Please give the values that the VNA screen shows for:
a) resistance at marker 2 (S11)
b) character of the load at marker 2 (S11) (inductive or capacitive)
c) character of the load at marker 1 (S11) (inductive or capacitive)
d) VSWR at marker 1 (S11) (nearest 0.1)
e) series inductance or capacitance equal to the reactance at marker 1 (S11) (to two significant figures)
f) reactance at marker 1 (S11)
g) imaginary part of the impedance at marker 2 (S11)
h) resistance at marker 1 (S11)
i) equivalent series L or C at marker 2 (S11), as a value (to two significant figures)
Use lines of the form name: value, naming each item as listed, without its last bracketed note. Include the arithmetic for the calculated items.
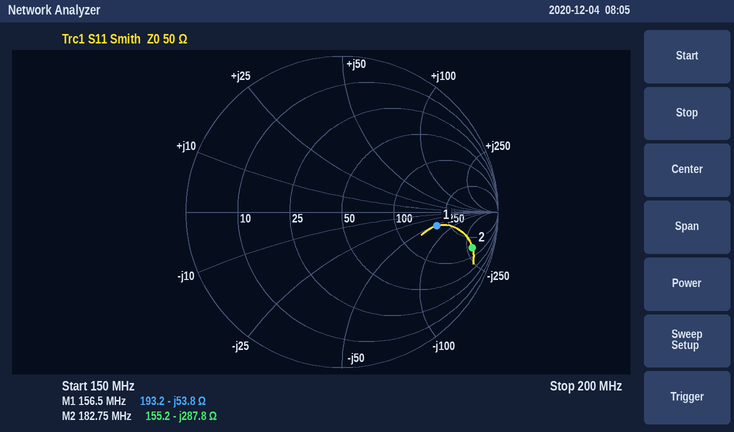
resistance at marker 2: 155.2 Ω
character of the load at marker 2 (S11): capacitive
character of the load at marker 1 (S11): capacitive
VSWR at marker 1 (S11): 4.2
series inductance or capacitance equal to the reactance at marker 1 (S11): C = 1/(2π × 156.5 MHz × 53.8 Ω) ≈ 19 pF
reactance at marker 1: -53.8 Ω
imaginary part of the impedance at marker 2: -287.8 Ω
resistance at marker 1: 193.2 Ω
equivalent series L or C at marker 2 (S11), as a value: C = 1/(2π × 182.75 MHz × 287.8 Ω) ≈ 3.0 pF
